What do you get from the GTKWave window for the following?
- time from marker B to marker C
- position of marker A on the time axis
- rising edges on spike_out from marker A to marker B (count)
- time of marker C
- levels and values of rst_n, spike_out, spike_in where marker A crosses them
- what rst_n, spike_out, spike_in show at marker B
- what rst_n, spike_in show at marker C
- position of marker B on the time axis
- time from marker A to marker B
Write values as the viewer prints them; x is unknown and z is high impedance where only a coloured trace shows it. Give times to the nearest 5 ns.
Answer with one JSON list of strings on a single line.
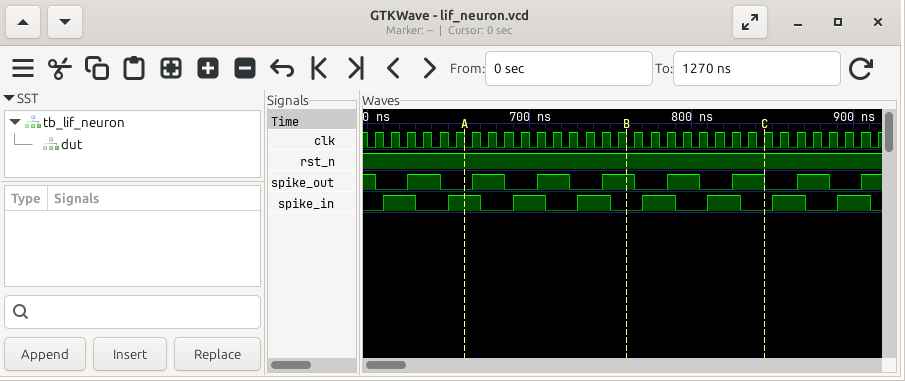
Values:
["85 ns", "660 ns", "3", "845 ns", "rst_n=1, spike_out=0, spike_in=1", "rst_n=1, spike_out=1, spike_in=0", "rst_n=1, spike_in=0", "760 ns", "100 ns"]
